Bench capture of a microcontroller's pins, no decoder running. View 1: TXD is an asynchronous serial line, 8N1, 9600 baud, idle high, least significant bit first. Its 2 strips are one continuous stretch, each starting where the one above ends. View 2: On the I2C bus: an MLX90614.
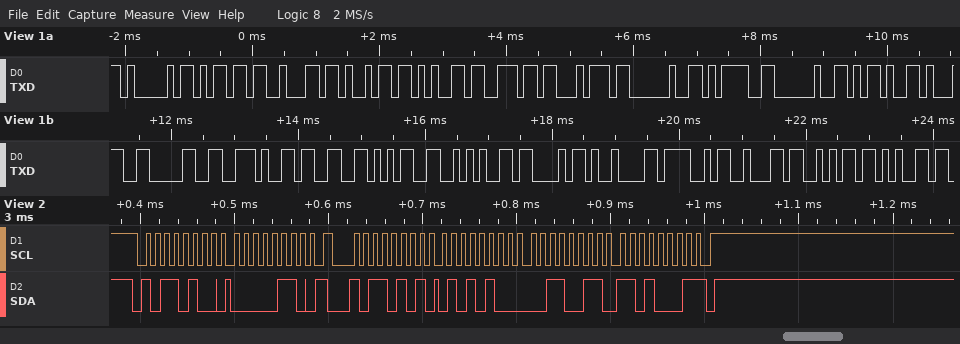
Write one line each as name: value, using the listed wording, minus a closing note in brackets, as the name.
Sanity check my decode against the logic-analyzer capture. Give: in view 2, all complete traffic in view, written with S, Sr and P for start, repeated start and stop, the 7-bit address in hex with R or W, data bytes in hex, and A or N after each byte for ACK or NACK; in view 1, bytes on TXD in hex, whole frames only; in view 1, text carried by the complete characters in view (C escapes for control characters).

in view 2, all complete traffic in view, written with S, Sr and P for start, repeated start and stop, the 7-bit address in hex with R or W, data bytes in hex, and A or N after each byte for ACK or NACK: S 5AW A 06 A Sr 5AR A 54 A 33 A D1 N P
in view 1, bytes on TXD in hex, whole frames only: 41 6D 62 69 65 6E 74 20 3D 20 2D 31 30 2E 33 35 2A 43 09 4F 62 6A 65
in view 1, text carried by the complete characters in view: "Ambient = -10.35*C\tObje"
